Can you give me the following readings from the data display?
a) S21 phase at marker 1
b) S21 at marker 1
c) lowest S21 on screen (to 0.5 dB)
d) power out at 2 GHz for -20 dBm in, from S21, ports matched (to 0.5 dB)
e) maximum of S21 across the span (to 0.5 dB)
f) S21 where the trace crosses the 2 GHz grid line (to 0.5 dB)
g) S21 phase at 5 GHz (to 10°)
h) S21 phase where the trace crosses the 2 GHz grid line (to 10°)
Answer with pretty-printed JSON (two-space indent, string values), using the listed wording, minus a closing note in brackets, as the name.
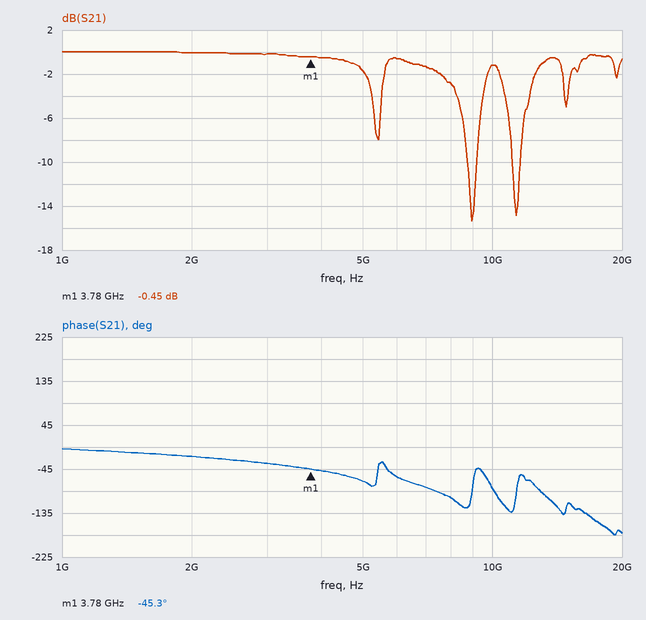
{
  "S21 phase at marker 1": "-45.3°",
  "S21 at marker 1": "-0.45 dB",
  "lowest S21 on screen": "-15.5 dB",
  "power out at 2 GHz for -20 dBm in, from S21, ports matched": "-20.0 dBm",
  "maximum of S21 across the span": "0.0 dB",
  "S21 where the trace crosses the 2 GHz grid line": "0.0 dB",
  "S21 phase at 5 GHz": "-70°",
  "S21 phase where the trace crosses the 2 GHz grid line": "-20°"
}
